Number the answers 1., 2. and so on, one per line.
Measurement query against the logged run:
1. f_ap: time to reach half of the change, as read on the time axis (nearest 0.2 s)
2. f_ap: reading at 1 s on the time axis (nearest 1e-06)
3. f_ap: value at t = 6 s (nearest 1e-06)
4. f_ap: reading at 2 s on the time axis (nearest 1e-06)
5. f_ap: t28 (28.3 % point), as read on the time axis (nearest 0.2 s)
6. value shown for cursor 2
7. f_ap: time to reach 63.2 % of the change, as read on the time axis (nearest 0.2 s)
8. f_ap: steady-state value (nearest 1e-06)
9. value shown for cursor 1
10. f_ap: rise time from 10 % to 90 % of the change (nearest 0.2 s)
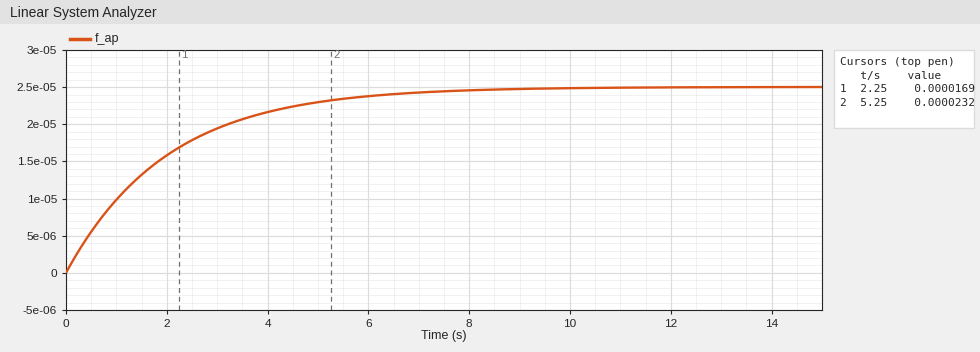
1. 1.4 s
2. 0.000010
3. 0.000024
4. 0.000016
5. 0.6 s
6. 0.0000232
7. 2.0 s
8. 0.000025
9. 0.0000169
10. 4.4 s
